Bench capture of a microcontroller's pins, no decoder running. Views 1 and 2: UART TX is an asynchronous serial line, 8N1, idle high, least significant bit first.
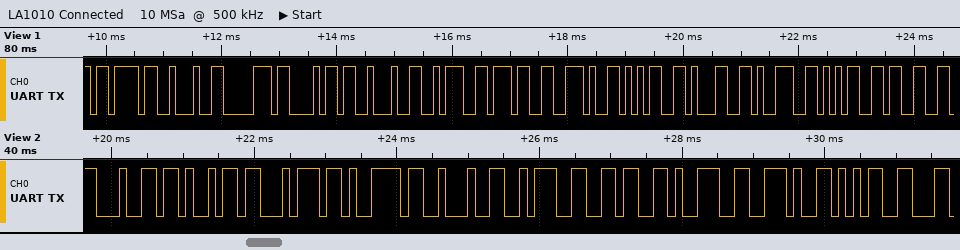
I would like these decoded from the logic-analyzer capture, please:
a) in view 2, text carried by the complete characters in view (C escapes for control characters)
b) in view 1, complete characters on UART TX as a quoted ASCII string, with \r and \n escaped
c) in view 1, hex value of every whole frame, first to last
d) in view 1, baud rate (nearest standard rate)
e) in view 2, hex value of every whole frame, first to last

"dity\":69.5"
"{\"ph\":7.51953"
7B 22 70 68 22 3A 37 2E 35 31 39 35 33
9600 baud
0x64 0x69 0x74 0x79 0x22 0x3A 0x36 0x39 0x2E 0x35
